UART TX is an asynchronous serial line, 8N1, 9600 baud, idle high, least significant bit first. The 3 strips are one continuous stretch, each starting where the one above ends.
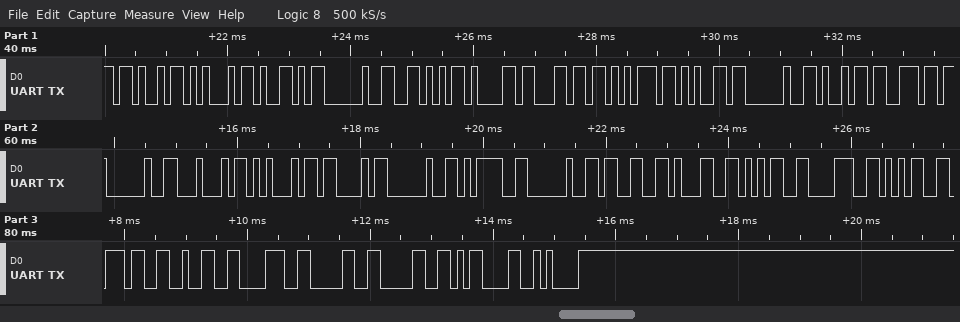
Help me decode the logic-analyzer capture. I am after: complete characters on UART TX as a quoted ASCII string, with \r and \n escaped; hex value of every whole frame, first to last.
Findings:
"KEY Value in DEC = 3158572800\r\n"
4B 45 59 20 56 61 6C 75 65 20 69 6E 20 44 45 43 20 3D 20 33 31 35 38 35 37 32 38 30 30 0D 0A
